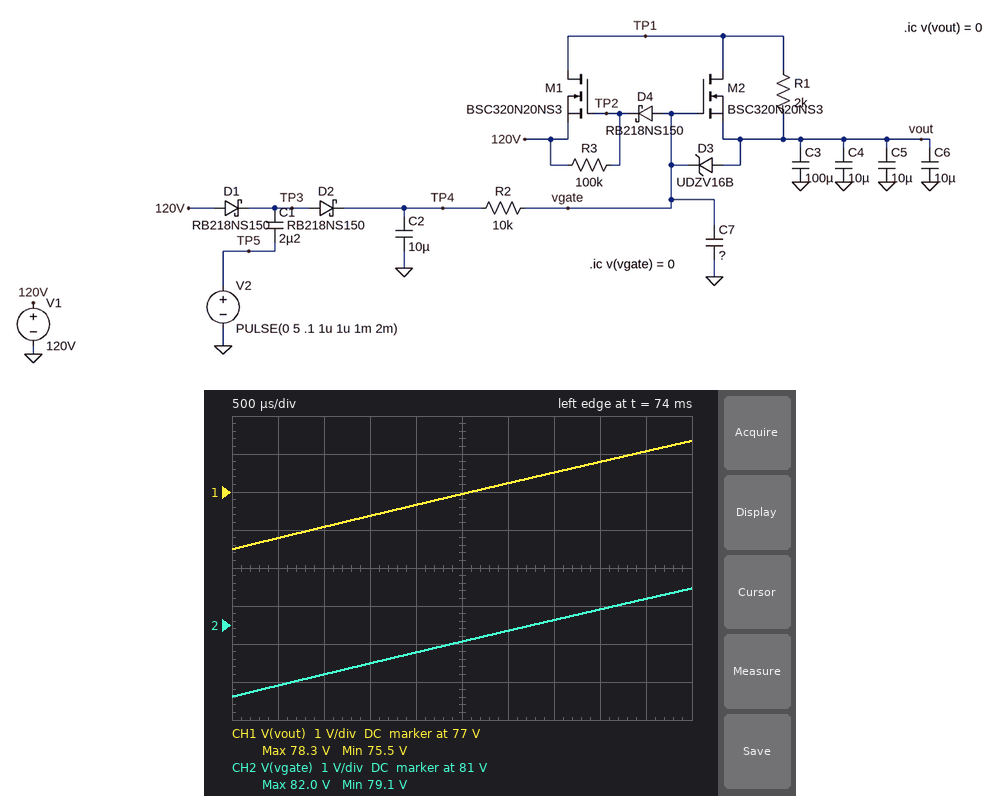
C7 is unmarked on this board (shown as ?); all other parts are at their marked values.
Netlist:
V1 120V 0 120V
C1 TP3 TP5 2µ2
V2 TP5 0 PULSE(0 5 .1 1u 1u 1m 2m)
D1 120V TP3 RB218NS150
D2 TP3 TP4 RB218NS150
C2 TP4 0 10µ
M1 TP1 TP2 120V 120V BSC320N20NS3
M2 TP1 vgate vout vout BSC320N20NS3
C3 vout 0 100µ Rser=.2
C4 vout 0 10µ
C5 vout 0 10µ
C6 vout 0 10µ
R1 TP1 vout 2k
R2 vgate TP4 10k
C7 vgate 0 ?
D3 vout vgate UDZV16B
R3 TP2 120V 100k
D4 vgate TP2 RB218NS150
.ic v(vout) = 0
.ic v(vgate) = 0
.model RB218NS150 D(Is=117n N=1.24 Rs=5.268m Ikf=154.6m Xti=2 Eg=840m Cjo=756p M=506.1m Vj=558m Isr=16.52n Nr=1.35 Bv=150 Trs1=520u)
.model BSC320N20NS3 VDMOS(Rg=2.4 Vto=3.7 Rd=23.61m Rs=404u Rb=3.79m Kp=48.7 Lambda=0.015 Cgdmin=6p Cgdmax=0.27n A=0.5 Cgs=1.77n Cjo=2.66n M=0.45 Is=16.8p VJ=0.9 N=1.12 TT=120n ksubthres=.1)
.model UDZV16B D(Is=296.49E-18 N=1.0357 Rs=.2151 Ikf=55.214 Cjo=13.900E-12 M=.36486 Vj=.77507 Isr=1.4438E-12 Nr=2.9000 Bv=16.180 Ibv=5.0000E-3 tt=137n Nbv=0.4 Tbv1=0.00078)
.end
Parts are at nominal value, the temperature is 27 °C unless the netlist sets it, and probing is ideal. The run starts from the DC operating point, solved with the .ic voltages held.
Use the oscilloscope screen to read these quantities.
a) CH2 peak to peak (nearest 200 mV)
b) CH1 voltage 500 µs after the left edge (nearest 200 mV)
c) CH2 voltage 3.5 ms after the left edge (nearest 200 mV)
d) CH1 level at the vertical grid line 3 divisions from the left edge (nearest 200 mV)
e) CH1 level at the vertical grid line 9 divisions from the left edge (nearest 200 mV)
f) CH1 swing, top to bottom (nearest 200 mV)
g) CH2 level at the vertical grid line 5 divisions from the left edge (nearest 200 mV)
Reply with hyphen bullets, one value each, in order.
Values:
- 2.8 V
- 75.8 V
- 81.2 V
- 76.4 V
- 78.0 V
- 2.8 V
- 80.6 V
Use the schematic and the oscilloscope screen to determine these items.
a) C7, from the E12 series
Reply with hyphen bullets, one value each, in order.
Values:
- 6.8 µF
